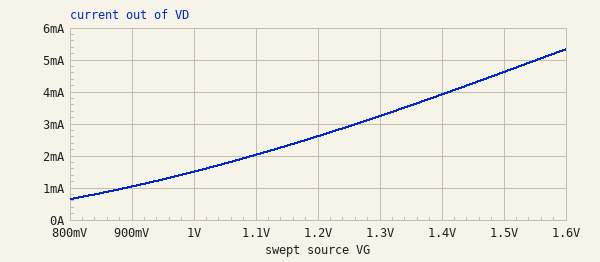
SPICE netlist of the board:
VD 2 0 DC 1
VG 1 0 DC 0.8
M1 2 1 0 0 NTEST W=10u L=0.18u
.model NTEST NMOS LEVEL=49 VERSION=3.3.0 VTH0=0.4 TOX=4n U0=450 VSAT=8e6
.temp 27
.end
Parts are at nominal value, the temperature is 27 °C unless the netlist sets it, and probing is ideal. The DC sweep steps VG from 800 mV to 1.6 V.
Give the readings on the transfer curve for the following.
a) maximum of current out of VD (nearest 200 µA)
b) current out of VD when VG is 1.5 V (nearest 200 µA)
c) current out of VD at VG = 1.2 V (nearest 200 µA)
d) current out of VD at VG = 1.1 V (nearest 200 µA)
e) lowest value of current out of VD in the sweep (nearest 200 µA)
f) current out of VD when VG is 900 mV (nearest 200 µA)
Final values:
5.4 mA
4.6 mA
2.6 mA
2.0 mA
600 µA
1.0 mA
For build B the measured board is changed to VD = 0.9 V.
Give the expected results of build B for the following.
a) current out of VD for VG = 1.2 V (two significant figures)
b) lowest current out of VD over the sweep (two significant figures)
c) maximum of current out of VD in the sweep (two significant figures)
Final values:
2.6 mA
640 µA
5.2 mA
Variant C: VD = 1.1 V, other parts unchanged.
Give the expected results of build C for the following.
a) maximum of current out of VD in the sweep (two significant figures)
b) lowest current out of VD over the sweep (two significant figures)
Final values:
5.4 mA
660 µA
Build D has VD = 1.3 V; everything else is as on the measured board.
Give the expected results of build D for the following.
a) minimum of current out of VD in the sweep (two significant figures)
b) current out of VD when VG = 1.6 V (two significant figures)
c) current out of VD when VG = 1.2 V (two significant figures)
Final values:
680 µA
5.5 mA
2.7 mA
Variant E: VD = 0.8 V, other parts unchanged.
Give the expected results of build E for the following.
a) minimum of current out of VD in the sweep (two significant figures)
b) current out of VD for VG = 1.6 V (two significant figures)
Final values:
630 µA
5.0 mA
